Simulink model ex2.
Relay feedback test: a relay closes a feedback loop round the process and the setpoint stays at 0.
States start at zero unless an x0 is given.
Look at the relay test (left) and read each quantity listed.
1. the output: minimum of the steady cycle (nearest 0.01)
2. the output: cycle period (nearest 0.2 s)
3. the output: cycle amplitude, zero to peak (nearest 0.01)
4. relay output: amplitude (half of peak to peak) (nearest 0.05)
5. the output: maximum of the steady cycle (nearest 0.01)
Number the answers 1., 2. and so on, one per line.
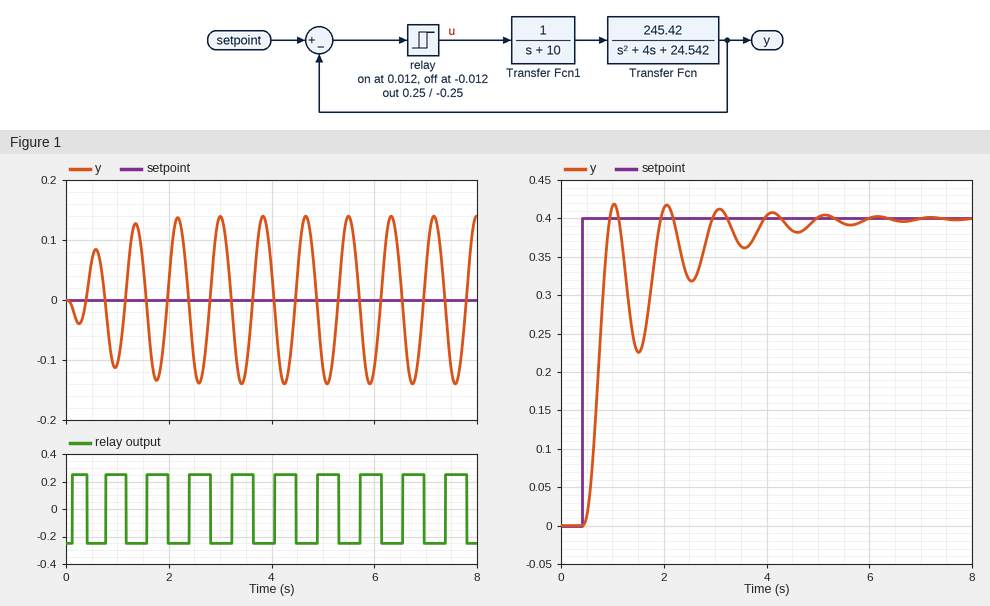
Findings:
1. -0.14
2. 0.8 s
3. 0.14
4. 0.25
5. 0.14
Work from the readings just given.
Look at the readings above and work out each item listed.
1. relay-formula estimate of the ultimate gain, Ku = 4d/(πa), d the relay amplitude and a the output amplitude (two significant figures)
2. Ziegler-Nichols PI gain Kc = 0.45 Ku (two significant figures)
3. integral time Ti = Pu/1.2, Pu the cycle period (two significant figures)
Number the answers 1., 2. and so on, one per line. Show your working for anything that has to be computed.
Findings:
1. 4 × 0.25 / (π × 0.14) = 2.3
2. 0.45 × 2.3 = 1.0
3. 0.8 / 1.2 = 0.67 s
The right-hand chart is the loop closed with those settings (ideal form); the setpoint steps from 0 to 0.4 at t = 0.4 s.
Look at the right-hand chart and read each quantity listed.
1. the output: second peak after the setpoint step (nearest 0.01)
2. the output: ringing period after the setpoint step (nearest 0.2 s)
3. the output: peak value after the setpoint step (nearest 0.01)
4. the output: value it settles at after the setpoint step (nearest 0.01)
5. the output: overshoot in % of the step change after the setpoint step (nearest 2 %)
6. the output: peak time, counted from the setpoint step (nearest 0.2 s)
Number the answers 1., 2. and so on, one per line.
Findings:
1. 0.42
2. 1.0 s
3. 0.42
4. 0.40
5. 4 %
6. 0.6 s
